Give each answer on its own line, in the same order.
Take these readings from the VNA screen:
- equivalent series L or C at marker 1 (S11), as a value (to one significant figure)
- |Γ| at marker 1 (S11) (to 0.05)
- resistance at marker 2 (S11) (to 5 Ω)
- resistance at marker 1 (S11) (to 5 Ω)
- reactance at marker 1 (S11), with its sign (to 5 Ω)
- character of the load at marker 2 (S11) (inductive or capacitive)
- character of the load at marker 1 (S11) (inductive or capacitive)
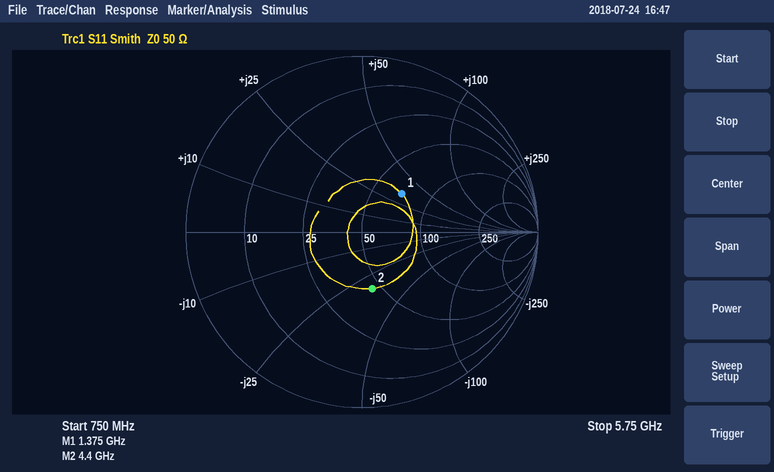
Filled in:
4 nH
0.30
45 Ω
70 Ω
+35 Ω
capacitive
inductive
